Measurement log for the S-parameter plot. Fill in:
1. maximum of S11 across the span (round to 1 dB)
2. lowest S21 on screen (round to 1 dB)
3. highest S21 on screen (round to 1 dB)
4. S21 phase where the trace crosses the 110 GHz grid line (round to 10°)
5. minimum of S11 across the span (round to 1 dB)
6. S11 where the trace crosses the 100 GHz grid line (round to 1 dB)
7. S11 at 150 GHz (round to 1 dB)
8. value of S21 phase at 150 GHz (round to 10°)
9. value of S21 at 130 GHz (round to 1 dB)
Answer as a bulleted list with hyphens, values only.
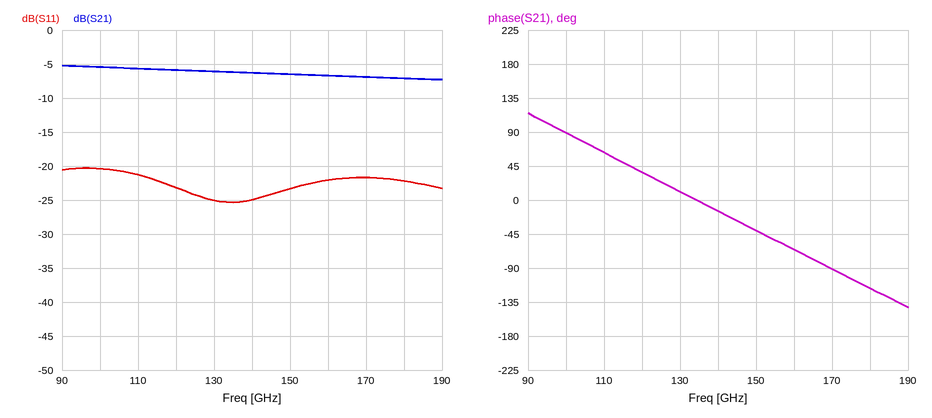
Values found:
- -20 dB
- -7 dB
- -5 dB
- 60°
- -25 dB
- -20 dB
- -23 dB
- -40°
- -6 dB
